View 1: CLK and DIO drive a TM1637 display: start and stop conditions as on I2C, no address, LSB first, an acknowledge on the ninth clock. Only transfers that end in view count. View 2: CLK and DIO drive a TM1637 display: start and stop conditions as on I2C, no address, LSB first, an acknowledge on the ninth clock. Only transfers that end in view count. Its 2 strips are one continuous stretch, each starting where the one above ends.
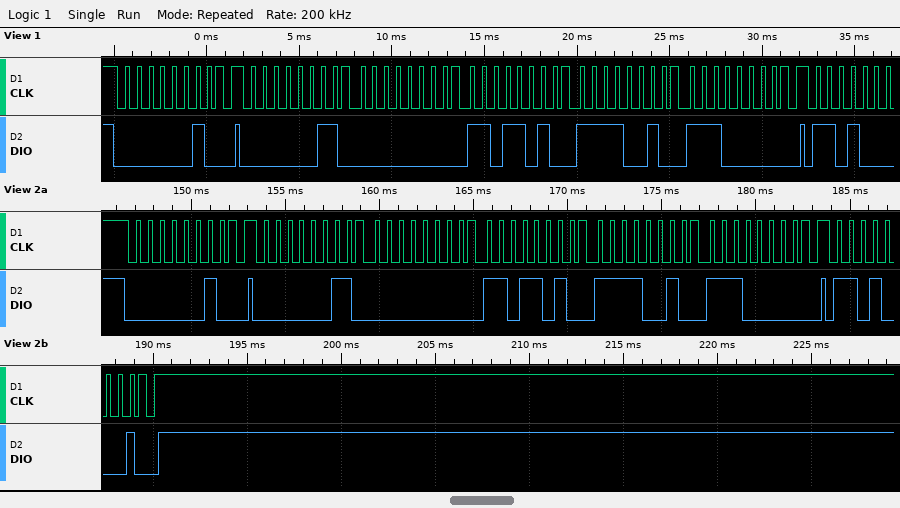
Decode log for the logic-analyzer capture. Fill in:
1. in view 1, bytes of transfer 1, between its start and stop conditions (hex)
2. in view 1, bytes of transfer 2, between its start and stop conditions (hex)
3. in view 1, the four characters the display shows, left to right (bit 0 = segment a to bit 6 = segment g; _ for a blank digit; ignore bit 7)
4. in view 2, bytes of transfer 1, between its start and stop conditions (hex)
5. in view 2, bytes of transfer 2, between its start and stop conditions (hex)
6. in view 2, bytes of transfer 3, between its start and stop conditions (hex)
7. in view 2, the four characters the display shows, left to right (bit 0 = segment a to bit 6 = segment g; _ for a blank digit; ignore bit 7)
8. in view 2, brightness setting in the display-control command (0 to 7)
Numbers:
40
C0 00 5B 4F 07
_237
40
C0 00 5B 4F 07
8B
_237
3
